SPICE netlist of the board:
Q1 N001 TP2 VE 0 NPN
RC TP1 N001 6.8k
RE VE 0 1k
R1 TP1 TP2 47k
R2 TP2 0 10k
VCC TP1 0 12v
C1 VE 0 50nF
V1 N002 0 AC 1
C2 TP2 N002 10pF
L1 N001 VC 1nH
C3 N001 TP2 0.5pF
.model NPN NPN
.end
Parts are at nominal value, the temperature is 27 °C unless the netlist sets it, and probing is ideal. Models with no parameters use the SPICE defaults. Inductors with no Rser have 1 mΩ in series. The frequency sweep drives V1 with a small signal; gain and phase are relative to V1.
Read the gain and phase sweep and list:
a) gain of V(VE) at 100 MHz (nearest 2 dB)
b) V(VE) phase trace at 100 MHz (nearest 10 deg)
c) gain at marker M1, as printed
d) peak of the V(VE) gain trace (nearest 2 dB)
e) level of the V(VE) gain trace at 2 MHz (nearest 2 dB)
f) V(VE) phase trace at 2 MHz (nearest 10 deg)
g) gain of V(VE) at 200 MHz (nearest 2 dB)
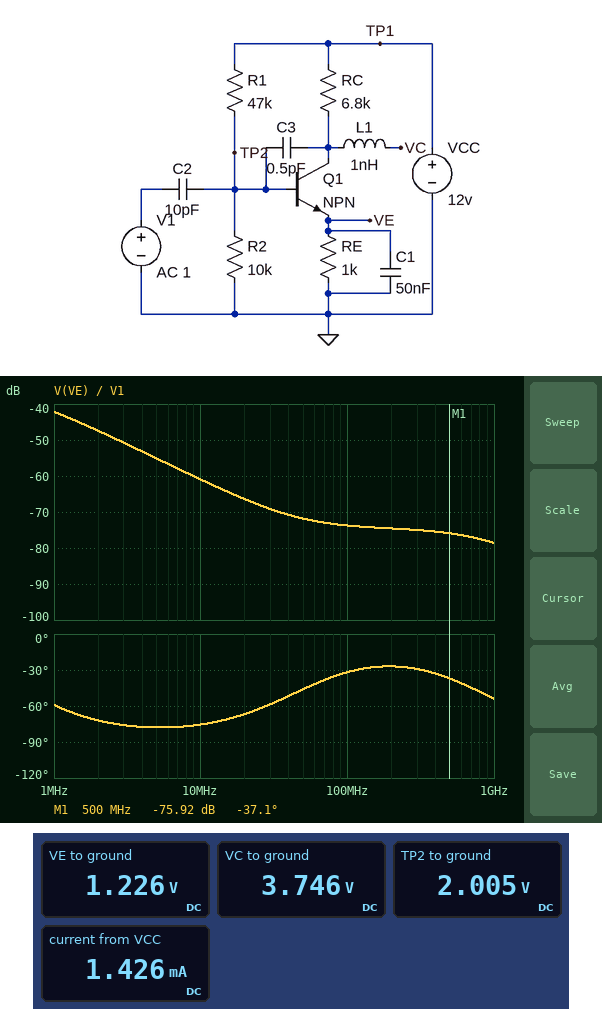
-74 dB
-30 deg
-75.92 dB
-42 dB
-48 dB
-70 deg
-74 dB
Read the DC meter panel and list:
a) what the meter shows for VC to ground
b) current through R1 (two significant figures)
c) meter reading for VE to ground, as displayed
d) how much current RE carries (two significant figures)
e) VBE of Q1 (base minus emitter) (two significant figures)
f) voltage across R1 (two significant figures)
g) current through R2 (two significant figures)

3.746 V
210 µA
1.226 V
1.2 mA
780 mV
10 V
200 µA
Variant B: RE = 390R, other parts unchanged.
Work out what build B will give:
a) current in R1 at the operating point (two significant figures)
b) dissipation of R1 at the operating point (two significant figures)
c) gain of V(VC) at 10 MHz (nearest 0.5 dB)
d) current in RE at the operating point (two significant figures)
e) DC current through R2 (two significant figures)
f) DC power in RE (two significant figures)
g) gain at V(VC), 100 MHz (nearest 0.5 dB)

220 µA
2.4 mW
-12.0 dB
1.7 mA
150 µA
1.2 mW
7.5 dB
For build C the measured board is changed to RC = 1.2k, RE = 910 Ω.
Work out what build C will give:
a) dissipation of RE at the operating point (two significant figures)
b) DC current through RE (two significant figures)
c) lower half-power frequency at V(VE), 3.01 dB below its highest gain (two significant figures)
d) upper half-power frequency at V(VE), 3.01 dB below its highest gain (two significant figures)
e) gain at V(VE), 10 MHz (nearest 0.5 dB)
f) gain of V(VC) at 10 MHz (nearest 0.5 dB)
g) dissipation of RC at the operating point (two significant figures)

1.6 mW
1.3 mA
34 kHz
2.5 MHz
-48.5 dB
23.0 dB
2.1 mW
